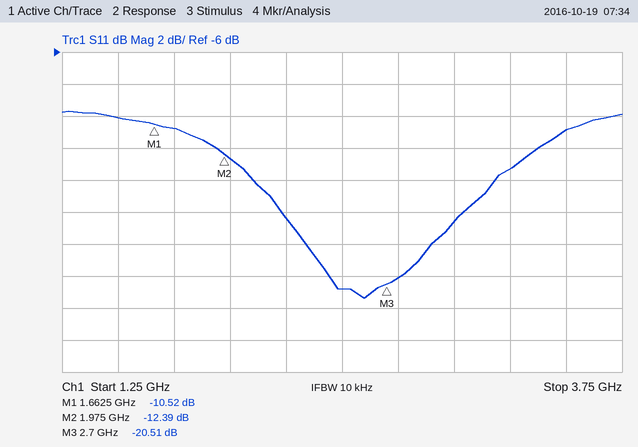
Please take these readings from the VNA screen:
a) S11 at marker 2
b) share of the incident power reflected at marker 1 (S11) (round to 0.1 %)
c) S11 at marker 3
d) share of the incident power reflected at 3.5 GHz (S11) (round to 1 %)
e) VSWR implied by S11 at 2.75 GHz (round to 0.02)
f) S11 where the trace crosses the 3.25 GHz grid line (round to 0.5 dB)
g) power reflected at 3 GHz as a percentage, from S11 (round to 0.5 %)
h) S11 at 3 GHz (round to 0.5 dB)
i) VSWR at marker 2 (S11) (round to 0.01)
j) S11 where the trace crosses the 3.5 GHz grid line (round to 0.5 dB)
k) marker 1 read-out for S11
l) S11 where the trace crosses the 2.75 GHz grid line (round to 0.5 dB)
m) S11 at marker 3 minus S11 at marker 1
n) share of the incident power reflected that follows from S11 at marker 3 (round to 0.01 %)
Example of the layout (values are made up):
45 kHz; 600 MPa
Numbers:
-12.39 dB; 8.9 %; -20.51 dB; 8 %; 1.22; -13.5 dB; 2.0 %; -16.5 dB; 1.63; -11.0 dB; -10.52 dB; -20.0 dB; -9.99 dB; 0.89 %
